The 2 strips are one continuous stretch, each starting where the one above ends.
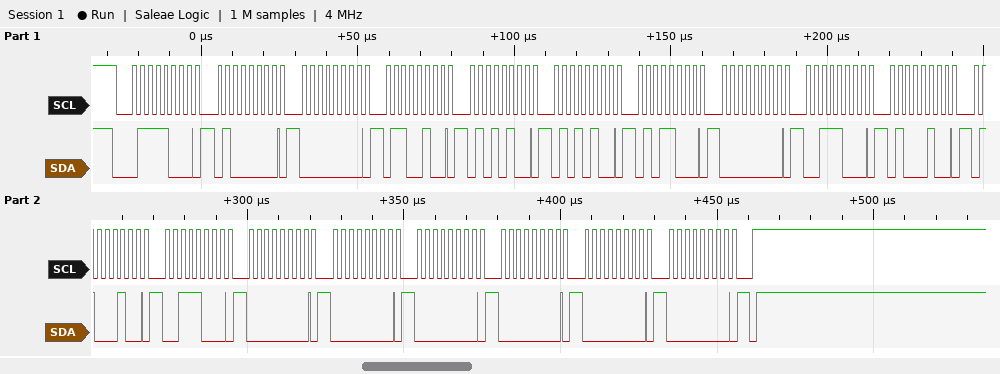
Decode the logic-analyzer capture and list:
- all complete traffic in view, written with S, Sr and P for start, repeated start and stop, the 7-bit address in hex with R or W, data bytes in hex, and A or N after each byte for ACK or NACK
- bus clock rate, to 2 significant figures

S 3CW A 40 A 00 A 64 A 54 A 54 A 58 A 00 A 38 A 44 A 44 A 38 A 00 A 00 A 00 A 00 A 00 A 00 A P
400 kHz
